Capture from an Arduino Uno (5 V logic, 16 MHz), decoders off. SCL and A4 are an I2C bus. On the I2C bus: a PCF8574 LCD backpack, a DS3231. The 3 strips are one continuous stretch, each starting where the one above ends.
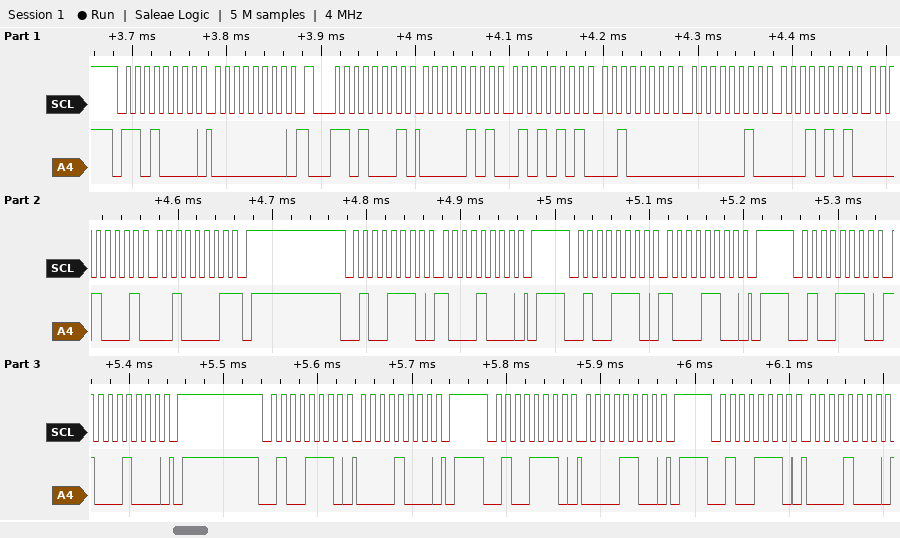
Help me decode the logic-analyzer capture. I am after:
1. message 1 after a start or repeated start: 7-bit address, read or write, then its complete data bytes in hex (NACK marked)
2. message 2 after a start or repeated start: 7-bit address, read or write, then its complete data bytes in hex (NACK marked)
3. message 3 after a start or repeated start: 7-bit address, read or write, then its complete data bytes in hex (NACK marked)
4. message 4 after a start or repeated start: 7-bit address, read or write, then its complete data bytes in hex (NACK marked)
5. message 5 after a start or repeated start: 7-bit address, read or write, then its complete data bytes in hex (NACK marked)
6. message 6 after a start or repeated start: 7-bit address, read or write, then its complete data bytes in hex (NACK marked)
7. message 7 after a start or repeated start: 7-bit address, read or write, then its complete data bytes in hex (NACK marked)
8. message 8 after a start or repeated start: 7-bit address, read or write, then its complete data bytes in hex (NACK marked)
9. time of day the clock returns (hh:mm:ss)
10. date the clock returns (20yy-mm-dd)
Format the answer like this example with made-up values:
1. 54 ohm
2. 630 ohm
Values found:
1. 0x68 write: 00
2. 0x68 read: 05 55 20 02 15 11 21 NACK
3. 0x27 write: 88
4. 0x27 write: 8C
5. 0x27 write: 88
6. 0x27 write: 08
7. 0x27 write: 0C
8. 0x27 write: 08
9. 20:55:05
10. 2021-11-15
